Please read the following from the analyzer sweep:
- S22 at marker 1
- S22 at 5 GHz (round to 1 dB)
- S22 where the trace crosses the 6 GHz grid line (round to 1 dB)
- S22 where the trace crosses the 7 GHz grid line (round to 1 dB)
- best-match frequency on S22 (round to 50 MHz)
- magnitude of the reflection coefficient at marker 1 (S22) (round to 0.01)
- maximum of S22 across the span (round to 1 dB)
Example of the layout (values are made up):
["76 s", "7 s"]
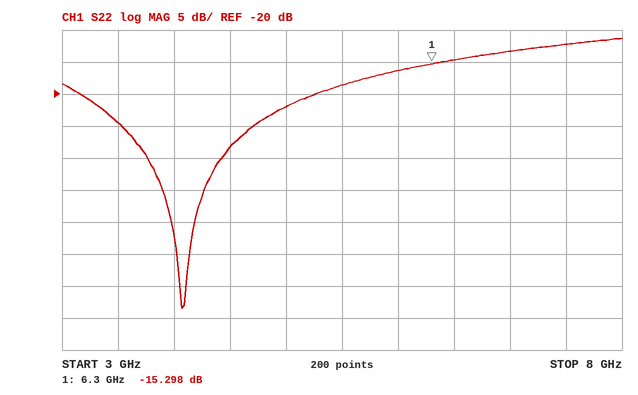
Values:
["-15.298 dB", "-22 dB", "-16 dB", "-13 dB", "4.05 GHz", "0.17", "-11 dB"]
